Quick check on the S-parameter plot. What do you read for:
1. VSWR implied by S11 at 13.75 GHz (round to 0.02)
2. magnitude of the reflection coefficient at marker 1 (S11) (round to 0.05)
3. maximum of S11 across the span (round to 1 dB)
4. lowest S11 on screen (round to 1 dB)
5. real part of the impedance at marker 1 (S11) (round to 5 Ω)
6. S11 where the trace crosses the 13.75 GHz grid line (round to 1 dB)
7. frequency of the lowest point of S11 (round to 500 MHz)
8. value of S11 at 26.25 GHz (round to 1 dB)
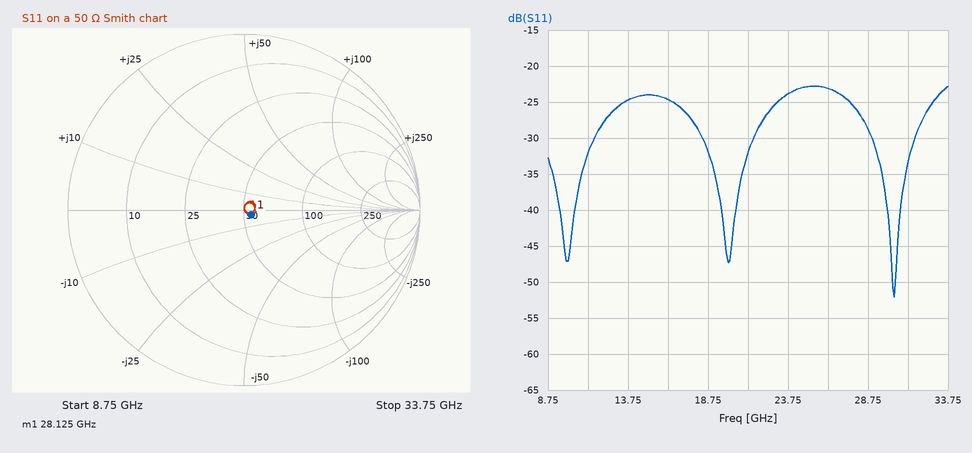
1.12
0.05
-23 dB
-52 dB
55 Ω
-25 dB
30.5 GHz
-23 dB
